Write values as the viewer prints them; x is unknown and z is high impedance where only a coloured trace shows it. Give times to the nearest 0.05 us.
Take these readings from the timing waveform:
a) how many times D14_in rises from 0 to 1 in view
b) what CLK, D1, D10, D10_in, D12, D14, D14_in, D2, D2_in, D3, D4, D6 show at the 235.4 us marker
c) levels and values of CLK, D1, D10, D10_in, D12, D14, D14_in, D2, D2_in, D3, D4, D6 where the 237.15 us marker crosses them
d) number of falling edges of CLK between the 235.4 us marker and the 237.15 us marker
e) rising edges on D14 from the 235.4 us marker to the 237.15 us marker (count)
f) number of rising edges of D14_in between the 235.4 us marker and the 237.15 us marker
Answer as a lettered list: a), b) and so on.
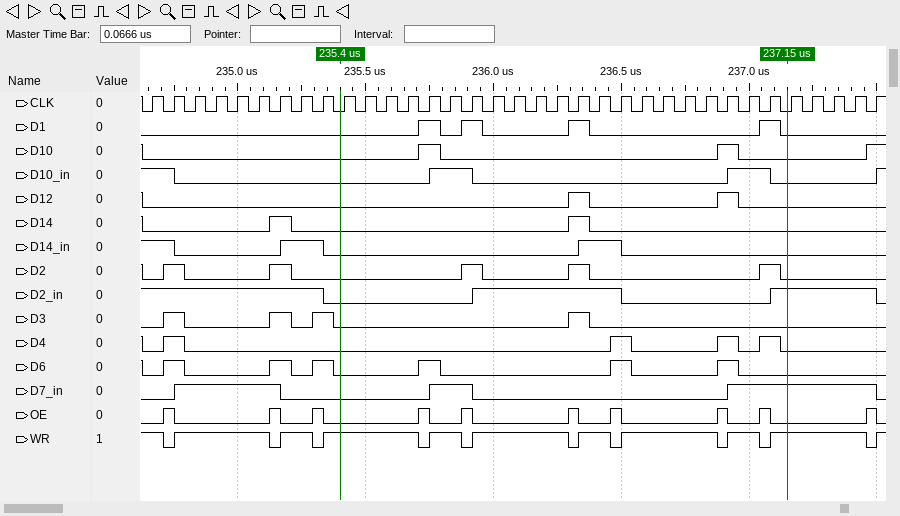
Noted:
a) 2
b) CLK=0, D1=0, D10=0, D10_in=0, D12=0, D14=0, D14_in=0, D2=0, D2_in=0, D3=0, D4=0, D6=0
c) CLK=0, D1=0, D10=0, D10_in=0, D12=0, D14=0, D14_in=0, D2=0, D2_in=1, D3=0, D4=0, D6=0
d) 21
e) 1
f) 1
